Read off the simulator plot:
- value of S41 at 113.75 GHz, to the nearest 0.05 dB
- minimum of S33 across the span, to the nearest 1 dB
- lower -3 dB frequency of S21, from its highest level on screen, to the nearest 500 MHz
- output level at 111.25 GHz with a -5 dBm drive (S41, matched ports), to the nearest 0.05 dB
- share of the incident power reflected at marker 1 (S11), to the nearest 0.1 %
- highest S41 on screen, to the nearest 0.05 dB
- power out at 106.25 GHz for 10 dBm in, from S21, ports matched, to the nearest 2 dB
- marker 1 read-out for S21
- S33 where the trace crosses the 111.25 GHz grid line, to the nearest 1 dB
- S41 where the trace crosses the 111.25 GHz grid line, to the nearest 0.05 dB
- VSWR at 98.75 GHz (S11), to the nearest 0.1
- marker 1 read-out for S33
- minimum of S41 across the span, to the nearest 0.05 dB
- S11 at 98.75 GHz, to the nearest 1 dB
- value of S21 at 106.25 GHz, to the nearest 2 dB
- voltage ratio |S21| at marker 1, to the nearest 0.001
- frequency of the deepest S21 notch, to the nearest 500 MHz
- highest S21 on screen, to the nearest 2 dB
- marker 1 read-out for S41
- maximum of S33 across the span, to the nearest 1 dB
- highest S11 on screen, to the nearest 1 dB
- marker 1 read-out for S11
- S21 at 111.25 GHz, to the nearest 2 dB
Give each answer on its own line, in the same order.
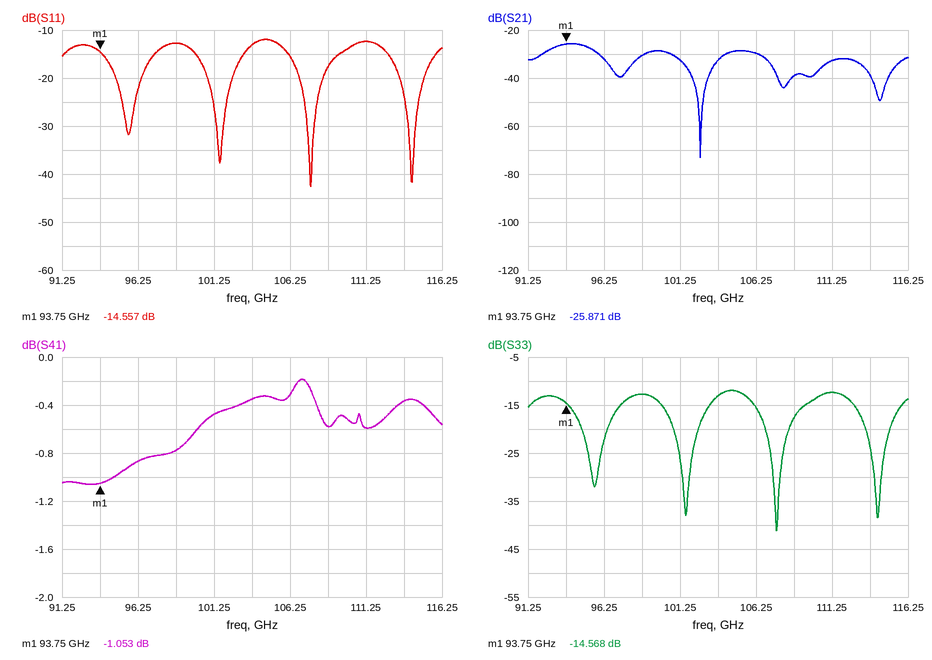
-0.35 dB
-41 dB
92.5 GHz
-5.60 dBm
3.5 %
-0.20 dB
-20 dBm
-25.871 dB
-12 dB
-0.60 dB
1.6
-14.568 dB
-1.05 dB
-13 dB
-30 dB
0.051
102.5 GHz
-26 dB
-1.053 dB
-12 dB
-12 dB
-14.557 dB
-32 dB
